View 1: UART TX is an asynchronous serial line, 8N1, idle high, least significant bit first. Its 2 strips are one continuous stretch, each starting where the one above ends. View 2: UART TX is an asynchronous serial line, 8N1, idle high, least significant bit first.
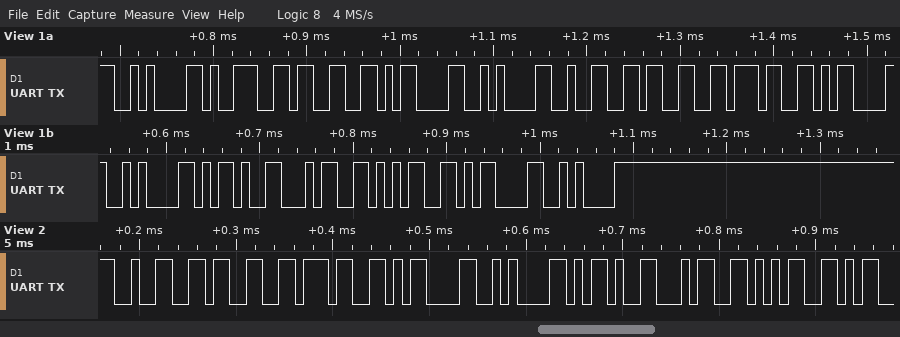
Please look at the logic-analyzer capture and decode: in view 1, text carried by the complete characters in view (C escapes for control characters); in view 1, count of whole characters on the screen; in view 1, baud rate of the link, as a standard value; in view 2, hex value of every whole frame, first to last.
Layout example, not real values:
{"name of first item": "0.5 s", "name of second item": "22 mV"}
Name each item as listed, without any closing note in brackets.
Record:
{"in view 1, text carried by the complete characters in view": "\"\\n93\\r\\n237\\r\\n-45\\r\\n\"", "in view 1, count of whole characters on the screen": "15", "in view 1, baud rate of the link, as a standard value": "115200 baud", "in view 2, hex value of every whole frame, first to last": "0x32 0x33 0x37 0x0D 0x0A 0x2D 0x34 0x35"}
